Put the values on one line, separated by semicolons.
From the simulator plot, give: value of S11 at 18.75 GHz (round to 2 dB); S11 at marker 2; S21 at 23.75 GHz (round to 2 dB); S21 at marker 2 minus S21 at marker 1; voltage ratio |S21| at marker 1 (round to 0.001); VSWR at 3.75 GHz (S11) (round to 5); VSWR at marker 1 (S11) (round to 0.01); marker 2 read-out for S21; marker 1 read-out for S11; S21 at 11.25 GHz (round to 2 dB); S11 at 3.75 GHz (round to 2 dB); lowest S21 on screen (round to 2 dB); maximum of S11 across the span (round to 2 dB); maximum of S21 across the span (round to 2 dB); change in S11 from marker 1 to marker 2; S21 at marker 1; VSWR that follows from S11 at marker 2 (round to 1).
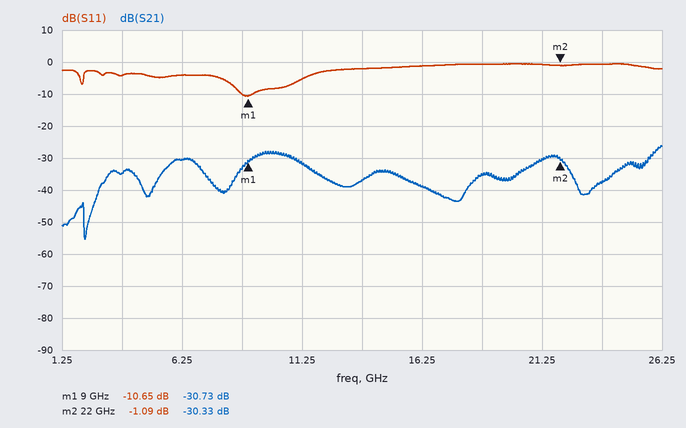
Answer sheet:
0 dB; -1.09 dB; -38 dB; 0.40 dB; 0.029; 5; 1.83; -30.33 dB; -10.65 dB; -32 dB; -4 dB; -56 dB; 0 dB; -26 dB; 9.56 dB; -30.73 dB; 16
